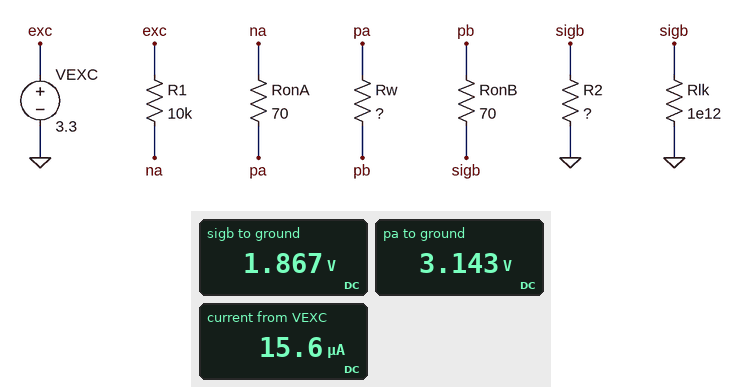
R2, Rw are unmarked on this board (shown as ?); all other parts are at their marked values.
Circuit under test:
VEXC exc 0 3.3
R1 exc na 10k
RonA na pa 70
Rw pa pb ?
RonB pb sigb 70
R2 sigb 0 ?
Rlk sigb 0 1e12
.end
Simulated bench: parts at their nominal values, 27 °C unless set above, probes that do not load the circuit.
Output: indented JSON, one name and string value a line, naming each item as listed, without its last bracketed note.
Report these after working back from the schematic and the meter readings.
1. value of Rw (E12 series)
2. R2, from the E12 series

{
  "value of Rw": "82 kΩ",
  "R2, from the E12 series": "120 kΩ"
}
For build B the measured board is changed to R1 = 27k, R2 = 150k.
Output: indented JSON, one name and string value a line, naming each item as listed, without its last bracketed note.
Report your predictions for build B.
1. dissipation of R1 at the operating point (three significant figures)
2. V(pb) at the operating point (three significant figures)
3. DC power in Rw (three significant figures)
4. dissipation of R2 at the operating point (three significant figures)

{
  "dissipation of R1 at the operating point": "4.38 µW",
  "V(pb) at the operating point": "1.91 V",
  "DC power in Rw": "13.3 µW",
  "dissipation of R2 at the operating point": "24.3 µW"
}
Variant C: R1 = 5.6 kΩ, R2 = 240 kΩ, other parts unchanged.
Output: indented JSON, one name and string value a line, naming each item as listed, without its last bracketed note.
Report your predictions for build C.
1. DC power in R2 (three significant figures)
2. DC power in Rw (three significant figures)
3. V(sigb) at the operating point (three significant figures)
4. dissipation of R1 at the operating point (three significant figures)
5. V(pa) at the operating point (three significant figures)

{
  "DC power in R2": "24.3 µW",
  "DC power in Rw": "8.31 µW",
  "V(sigb) at the operating point": "2.42 V",
  "dissipation of R1 at the operating point": "568 nW",
  "V(pa) at the operating point": "3.24 V"
}
